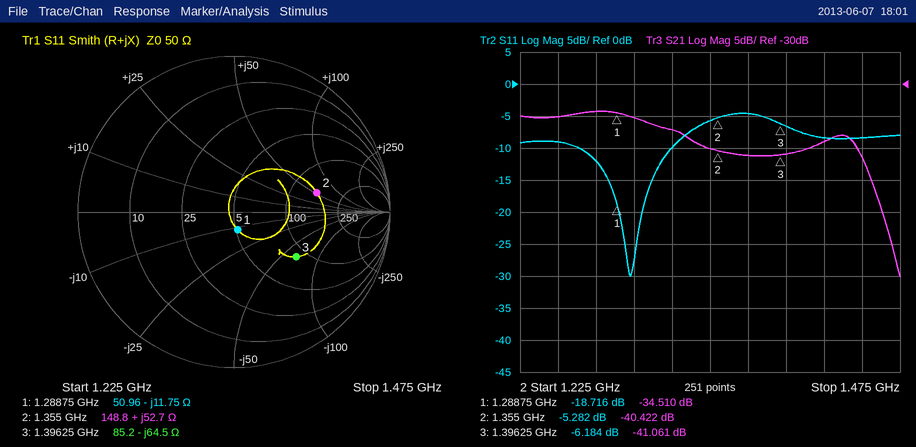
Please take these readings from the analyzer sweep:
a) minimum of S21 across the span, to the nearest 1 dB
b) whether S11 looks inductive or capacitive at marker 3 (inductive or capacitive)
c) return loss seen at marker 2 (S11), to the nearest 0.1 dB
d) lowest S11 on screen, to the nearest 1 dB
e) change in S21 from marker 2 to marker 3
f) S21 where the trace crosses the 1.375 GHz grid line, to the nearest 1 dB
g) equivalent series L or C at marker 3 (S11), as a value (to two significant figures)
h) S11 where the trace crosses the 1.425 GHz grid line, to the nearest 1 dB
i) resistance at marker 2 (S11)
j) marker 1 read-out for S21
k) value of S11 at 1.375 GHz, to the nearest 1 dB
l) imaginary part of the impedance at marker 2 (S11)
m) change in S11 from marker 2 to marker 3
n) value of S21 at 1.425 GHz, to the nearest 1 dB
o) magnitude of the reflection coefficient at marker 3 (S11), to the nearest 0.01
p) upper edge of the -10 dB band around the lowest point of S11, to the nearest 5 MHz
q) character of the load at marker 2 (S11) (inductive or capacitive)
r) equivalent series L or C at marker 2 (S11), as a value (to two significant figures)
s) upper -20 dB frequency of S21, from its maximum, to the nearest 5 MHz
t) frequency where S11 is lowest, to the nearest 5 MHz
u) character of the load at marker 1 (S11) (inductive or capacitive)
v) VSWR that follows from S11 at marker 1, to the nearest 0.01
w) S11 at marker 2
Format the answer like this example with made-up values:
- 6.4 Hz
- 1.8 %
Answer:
- -60 dB
- capacitive
- 5.3 dB
- -30 dB
- -0.639 dB
- -41 dB
- 1.8 pF
- -8 dB
- 148.8 Ω
- -34.510 dB
- -5 dB
- +52.7 Ω
- -0.902 dB
- -39 dB
- 0.49
- 1.325 GHz
- inductive
- 6.2 nH
- 1.470 GHz
- 1.300 GHz
- capacitive
- 1.26
- -5.282 dB
